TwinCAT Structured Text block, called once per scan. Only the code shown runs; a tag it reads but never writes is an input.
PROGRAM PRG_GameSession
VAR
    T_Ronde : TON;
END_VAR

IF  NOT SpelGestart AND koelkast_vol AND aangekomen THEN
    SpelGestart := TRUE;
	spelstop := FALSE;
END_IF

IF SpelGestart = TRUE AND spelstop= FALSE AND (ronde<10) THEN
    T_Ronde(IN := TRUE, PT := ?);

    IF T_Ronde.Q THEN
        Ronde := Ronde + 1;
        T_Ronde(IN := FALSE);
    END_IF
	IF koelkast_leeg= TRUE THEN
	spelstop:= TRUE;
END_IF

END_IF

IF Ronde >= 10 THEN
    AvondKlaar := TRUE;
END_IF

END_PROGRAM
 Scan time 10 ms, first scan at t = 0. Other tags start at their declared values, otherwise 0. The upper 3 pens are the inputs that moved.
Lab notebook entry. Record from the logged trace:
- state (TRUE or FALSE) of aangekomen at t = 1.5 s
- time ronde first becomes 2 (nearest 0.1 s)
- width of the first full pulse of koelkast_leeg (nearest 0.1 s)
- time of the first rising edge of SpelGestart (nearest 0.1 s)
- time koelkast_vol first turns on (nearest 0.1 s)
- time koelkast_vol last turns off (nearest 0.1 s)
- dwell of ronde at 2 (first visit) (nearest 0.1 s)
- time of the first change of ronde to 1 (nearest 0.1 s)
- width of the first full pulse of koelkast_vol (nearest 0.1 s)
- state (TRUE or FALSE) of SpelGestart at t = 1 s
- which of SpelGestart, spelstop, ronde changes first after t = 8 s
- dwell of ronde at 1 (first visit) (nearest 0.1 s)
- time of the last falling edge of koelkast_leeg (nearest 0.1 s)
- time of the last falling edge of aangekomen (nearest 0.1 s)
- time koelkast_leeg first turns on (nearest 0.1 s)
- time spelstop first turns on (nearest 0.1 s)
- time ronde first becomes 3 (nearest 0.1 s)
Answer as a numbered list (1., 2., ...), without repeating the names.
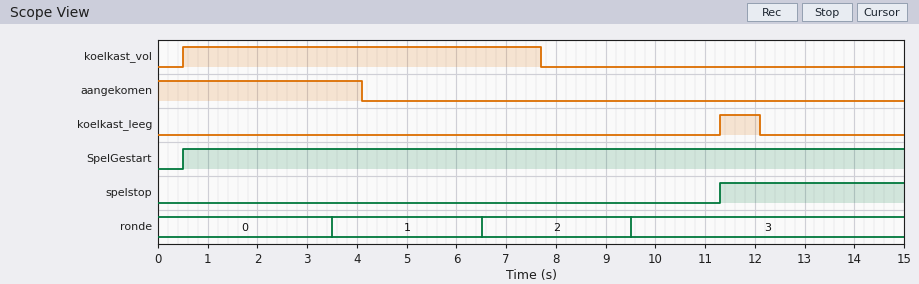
1. TRUE
2. 6.5 s
3. 0.8 s
4. 0.5 s
5. 0.5 s
6. 7.7 s
7. 3.0 s
8. 3.5 s
9. 7.2 s
10. TRUE
11. ronde
12. 3.0 s
13. 12.1 s
14. 4.1 s
15. 11.3 s
16. 11.3 s
17. 9.5 s
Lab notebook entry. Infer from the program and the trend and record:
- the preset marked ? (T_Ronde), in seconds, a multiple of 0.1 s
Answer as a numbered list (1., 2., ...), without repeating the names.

1. 3.0 s
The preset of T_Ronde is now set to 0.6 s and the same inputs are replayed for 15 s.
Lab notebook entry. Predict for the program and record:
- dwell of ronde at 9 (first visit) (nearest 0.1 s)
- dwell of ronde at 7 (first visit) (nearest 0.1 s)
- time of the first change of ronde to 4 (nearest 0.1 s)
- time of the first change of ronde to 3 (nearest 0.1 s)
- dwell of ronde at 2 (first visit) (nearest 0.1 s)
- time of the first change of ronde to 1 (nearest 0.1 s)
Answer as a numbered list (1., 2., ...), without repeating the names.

1. 0.6 s
2. 0.6 s
3. 2.9 s
4. 2.3 s
5. 0.6 s
6. 1.1 s
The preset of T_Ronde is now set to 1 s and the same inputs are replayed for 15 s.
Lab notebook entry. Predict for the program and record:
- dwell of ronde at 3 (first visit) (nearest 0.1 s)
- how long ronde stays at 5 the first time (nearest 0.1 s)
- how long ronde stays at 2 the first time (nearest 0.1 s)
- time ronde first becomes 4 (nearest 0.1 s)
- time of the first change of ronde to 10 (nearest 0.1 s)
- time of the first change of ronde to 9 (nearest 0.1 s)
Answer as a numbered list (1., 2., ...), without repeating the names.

1. 1.0 s
2. 1.0 s
3. 1.0 s
4. 4.5 s
5. 10.6 s
6. 9.6 s
